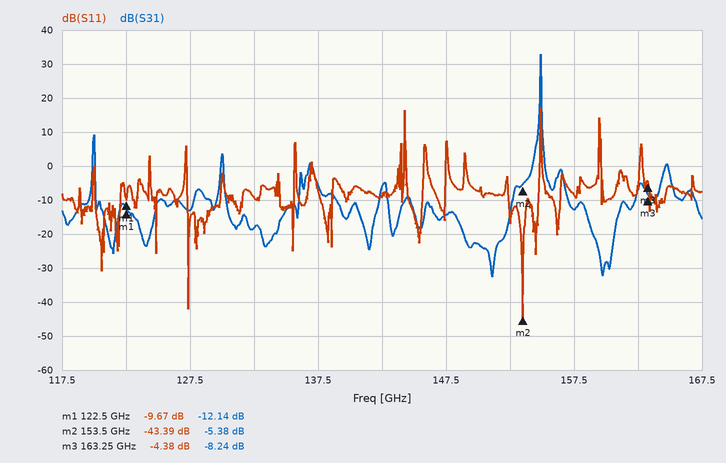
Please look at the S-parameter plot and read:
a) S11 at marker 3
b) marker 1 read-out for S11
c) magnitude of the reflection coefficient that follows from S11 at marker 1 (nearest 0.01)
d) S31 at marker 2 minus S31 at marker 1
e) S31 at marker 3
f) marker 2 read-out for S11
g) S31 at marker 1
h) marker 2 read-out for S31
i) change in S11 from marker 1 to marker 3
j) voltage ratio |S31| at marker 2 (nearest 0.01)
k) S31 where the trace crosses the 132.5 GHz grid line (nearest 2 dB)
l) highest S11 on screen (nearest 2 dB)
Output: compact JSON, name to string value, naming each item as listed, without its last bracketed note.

{"S11 at marker 3": "-4.38 dB", "marker 1 read-out for S11": "-9.67 dB", "magnitude of the reflection coefficient that follows from S11 at marker 1": "0.33", "S31 at marker 2 minus S31 at marker 1": "6.76 dB", "S31 at marker 3": "-8.24 dB", "marker 2 read-out for S11": "-43.39 dB", "S31 at marker 1": "-12.14 dB", "marker 2 read-out for S31": "-5.38 dB", "change in S11 from marker 1 to marker 3": "5.29 dB", "voltage ratio |S31| at marker 2": "0.54", "S31 where the trace crosses the 132.5 GHz grid line": "-18 dB", "highest S11 on screen": "18 dB"}
